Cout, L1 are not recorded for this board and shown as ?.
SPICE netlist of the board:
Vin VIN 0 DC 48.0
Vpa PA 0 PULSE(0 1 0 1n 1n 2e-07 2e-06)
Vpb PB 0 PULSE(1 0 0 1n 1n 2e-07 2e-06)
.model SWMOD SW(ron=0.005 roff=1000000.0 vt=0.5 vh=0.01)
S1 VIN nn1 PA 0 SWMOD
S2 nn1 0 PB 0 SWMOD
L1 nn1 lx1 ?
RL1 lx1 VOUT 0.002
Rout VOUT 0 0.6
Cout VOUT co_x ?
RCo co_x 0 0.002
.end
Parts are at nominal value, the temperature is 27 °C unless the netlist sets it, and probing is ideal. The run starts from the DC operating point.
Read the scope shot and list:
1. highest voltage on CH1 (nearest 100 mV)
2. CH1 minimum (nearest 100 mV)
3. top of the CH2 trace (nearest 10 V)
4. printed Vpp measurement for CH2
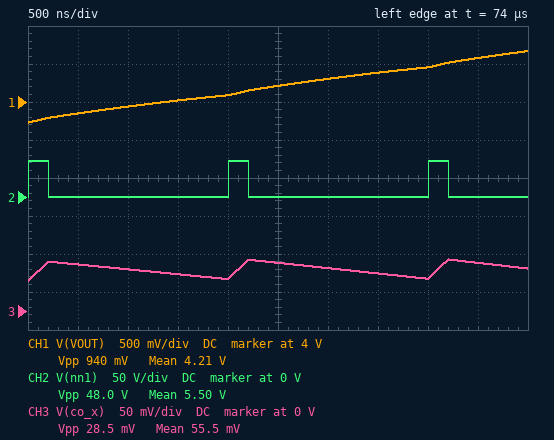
4.7 V
3.7 V
50 V
48.0 V
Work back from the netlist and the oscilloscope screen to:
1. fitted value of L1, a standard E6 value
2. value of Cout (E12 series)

680 nH
150 µF
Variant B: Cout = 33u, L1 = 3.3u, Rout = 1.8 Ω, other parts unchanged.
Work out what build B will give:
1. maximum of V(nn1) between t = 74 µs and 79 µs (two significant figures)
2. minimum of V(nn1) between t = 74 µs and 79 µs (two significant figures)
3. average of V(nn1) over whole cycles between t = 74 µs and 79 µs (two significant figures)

48 V
-51 mV
4.8 V
